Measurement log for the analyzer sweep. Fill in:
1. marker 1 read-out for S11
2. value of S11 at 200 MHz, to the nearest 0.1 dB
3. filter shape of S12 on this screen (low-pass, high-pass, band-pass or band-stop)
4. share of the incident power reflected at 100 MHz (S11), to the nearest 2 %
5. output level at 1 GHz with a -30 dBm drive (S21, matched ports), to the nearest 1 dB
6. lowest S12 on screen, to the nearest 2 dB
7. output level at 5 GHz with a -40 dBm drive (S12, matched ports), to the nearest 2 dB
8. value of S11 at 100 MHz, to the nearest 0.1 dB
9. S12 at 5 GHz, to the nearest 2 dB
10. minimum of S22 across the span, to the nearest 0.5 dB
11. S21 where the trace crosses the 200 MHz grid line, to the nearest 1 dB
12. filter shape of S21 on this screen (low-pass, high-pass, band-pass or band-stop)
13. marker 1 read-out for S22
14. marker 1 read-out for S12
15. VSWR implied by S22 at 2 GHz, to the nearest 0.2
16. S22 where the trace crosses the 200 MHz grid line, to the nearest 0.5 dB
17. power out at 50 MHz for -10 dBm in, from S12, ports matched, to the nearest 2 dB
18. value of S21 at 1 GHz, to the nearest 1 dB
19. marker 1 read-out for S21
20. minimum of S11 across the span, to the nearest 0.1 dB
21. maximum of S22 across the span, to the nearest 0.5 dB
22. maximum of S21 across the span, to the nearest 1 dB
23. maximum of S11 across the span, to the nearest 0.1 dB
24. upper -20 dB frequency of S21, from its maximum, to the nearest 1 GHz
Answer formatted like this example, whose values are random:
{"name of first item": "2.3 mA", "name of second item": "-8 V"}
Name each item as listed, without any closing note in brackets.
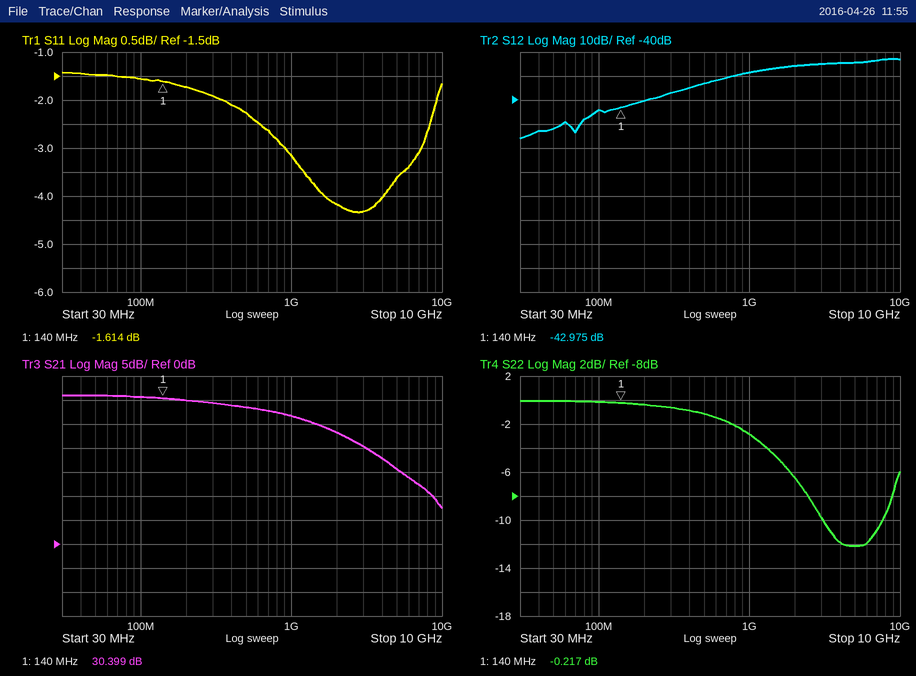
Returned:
{"marker 1 read-out for S11": "-1.614 dB", "value of S11 at 200 MHz, to the nearest 0.1 dB": "-1.7 dB", "filter shape of S12 on this screen": "high-pass", "share of the incident power reflected at 100 MHz (S11), to the nearest 2 %": "70 %", "output level at 1 GHz with a -30 dBm drive (S21, matched ports), to the nearest 1 dB": "-3 dBm", "lowest S12 on screen, to the nearest 2 dB": "-56 dB", "output level at 5 GHz with a -40 dBm drive (S12, matched ports), to the nearest 2 dB": "-64 dBm", "value of S11 at 100 MHz, to the nearest 0.1 dB": "-1.6 dB", "S12 at 5 GHz, to the nearest 2 dB": "-24 dB", "minimum of S22 across the span, to the nearest 0.5 dB": "-12.0 dB", "S21 where the trace crosses the 200 MHz grid line, to the nearest 1 dB": "30 dB", "filter shape of S21 on this screen": "low-pass", "marker 1 read-out for S22": "-0.217 dB", "marker 1 read-out for S12": "-42.975 dB", "VSWR implied by S22 at 2 GHz, to the nearest 0.2": "2.8", "S22 where the trace crosses the 200 MHz grid line, to the nearest 0.5 dB": "-0.5 dB", "power out at 50 MHz for -10 dBm in, from S12, ports matched, to the nearest 2 dB": "-62 dBm", "value of S21 at 1 GHz, to the nearest 1 dB": "27 dB", "marker 1 read-out for S21": "30.399 dB", "minimum of S11 across the span, to the nearest 0.1 dB": "-4.3 dB", "maximum of S22 across the span, to the nearest 0.5 dB": "0.0 dB", "maximum of S21 across the span, to the nearest 1 dB": "31 dB", "maximum of S11 across the span, to the nearest 0.1 dB": "-1.4 dB", "upper -20 dB frequency of S21, from its maximum, to the nearest 1 GHz": "8 GHz"}
